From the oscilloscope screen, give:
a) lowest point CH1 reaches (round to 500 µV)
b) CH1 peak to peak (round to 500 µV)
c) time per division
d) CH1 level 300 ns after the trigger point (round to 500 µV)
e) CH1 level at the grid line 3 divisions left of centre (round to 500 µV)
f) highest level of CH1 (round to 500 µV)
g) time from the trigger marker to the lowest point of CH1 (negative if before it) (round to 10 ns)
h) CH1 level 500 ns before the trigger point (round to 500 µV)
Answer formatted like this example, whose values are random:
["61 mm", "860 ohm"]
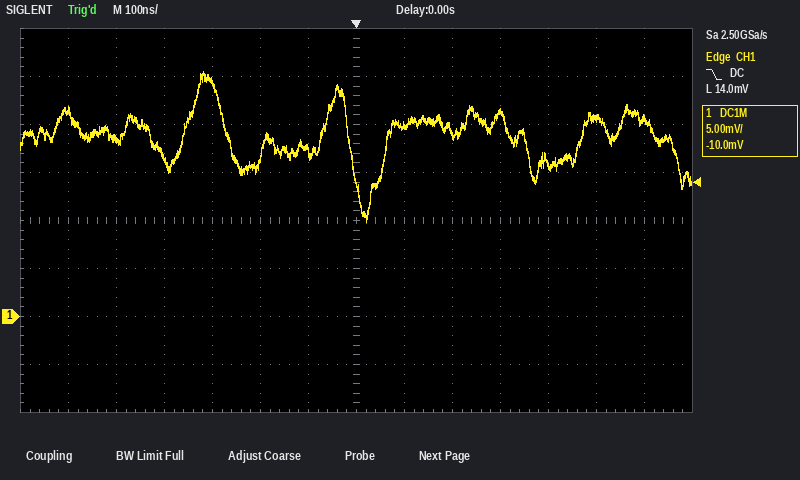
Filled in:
["10.0 mV", "15.5 mV", "100 ns", "21.5 mV", "24.5 mV", "25.5 mV", "+20 ns", "18.5 mV"]
